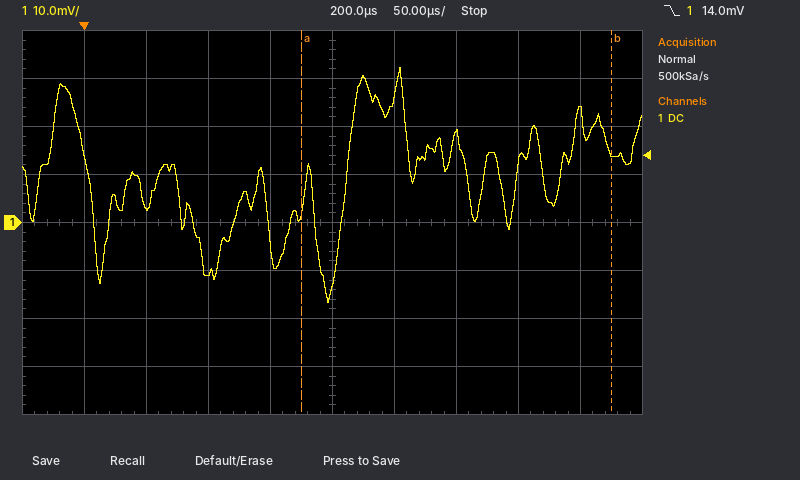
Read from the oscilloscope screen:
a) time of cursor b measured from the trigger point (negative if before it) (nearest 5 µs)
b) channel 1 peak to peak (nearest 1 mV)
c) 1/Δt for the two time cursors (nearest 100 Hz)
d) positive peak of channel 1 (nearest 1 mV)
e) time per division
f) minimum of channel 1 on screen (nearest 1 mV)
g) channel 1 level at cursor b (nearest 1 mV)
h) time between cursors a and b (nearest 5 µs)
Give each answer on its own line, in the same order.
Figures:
+425 µs
49 mV
4.0 kHz
32 mV
50 µs
-17 mV
15 mV
250 µs
